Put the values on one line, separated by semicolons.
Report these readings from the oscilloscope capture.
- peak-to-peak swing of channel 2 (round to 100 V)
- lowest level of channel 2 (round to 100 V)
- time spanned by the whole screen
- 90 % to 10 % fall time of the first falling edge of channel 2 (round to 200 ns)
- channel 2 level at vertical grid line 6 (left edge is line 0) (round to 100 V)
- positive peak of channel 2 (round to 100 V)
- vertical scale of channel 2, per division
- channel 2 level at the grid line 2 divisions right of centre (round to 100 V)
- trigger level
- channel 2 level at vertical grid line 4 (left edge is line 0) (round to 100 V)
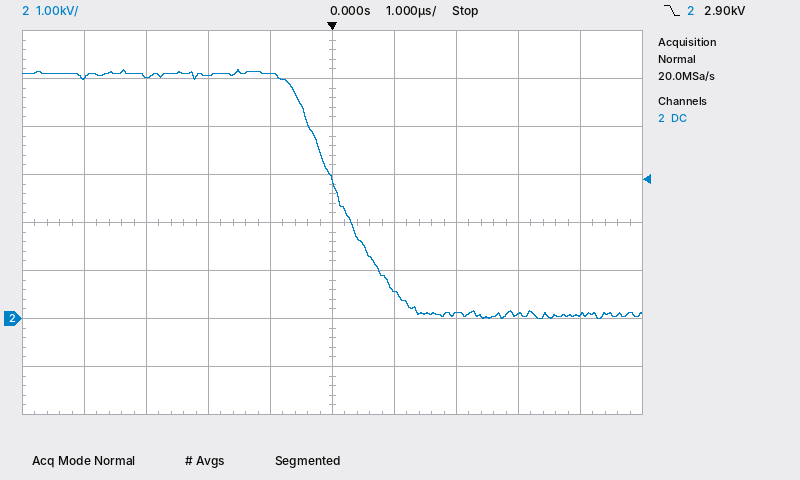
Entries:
5.2 kV; 0.0 kV; 10 µs; 1.6 µs; 600 V; 5.2 kV; 1 kV; 100 V; 2.90 kV; 5.1 kV
